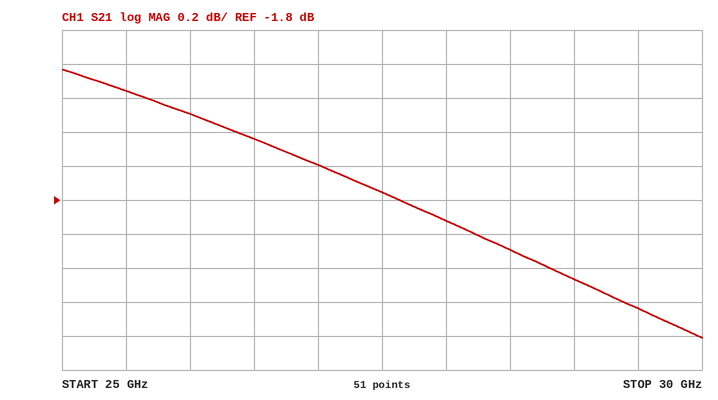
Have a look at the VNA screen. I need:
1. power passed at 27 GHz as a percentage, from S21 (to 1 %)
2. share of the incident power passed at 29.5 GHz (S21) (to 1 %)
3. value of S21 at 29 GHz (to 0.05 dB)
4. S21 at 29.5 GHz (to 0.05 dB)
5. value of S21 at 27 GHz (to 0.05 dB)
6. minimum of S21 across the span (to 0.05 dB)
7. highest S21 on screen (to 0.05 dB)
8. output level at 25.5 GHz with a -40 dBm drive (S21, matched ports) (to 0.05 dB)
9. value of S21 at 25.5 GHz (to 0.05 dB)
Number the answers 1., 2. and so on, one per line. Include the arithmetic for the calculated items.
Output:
1. 10^(-1.6/10) ≈ 69 %
2. 10^(-2.45/10) ≈ 57 %
3. -2.25 dB
4. -2.45 dB
5. -1.60 dB
6. -2.60 dB
7. -1.05 dB
8. -40 dBm + (-1.15 dB) = -41.15 dBm
9. -1.15 dB
